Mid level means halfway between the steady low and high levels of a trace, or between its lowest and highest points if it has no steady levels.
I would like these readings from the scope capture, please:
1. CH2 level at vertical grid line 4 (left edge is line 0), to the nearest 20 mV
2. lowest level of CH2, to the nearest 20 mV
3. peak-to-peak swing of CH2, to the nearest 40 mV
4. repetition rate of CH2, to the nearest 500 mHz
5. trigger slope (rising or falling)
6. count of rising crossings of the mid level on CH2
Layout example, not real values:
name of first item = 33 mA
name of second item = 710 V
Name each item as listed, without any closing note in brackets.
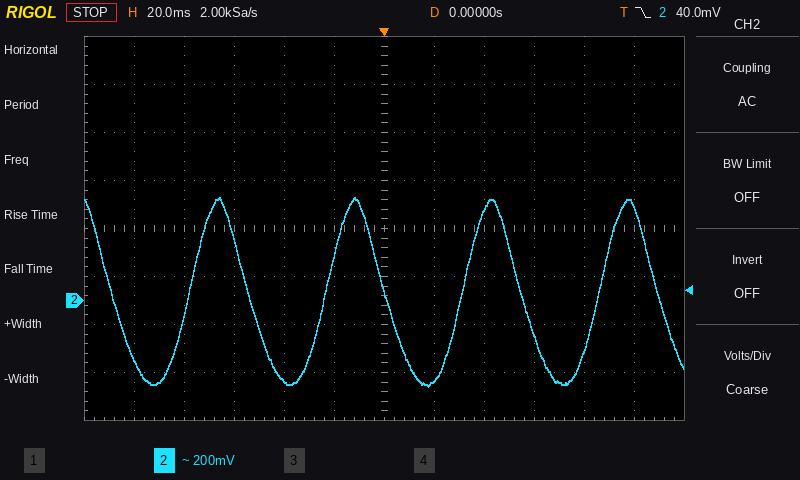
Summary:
CH2 level at vertical grid line 4 (left edge is line 0), to the nearest 20 mV = -340 mV
lowest level of CH2, to the nearest 20 mV = -360 mV
peak-to-peak swing of CH2, to the nearest 40 mV = 800 mV
repetition rate of CH2, to the nearest 500 mHz = 18.5 Hz
trigger slope = falling
count of rising crossings of the mid level on CH2 = 4
